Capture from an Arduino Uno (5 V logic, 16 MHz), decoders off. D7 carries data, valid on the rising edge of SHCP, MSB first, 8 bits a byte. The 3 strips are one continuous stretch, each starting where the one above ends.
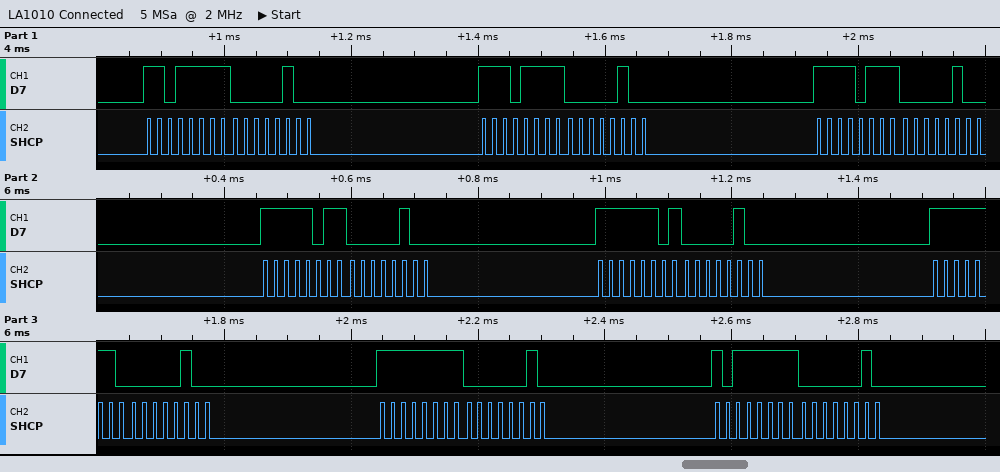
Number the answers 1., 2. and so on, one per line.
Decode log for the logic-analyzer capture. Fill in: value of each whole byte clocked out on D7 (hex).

1. DF 04 EF 04 F7 04 FB 04 FD 04 FE 04 FF 02 BF 02
